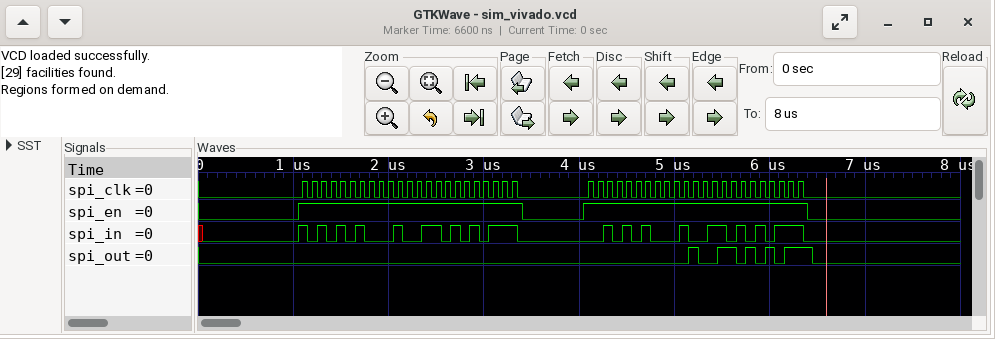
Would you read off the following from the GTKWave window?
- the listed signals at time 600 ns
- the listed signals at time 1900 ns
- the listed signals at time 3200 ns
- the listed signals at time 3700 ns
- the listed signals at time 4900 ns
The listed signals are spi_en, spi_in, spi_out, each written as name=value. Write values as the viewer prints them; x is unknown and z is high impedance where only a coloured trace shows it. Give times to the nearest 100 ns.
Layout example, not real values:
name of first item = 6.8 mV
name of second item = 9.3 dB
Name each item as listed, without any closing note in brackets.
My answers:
the listed signals at time 600 ns = spi_en=0, spi_in=0, spi_out=0
the listed signals at time 1900 ns = spi_en=1, spi_in=0, spi_out=0
the listed signals at time 3200 ns = spi_en=1, spi_in=1, spi_out=0
the listed signals at time 3700 ns = spi_en=0, spi_in=0, spi_out=0
the listed signals at time 4900 ns = spi_en=1, spi_in=0, spi_out=0
